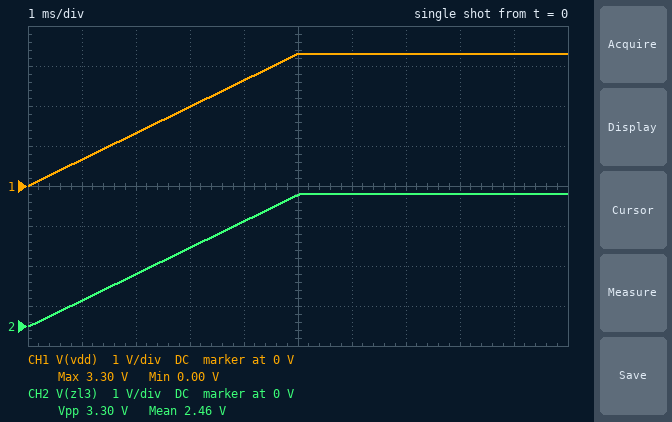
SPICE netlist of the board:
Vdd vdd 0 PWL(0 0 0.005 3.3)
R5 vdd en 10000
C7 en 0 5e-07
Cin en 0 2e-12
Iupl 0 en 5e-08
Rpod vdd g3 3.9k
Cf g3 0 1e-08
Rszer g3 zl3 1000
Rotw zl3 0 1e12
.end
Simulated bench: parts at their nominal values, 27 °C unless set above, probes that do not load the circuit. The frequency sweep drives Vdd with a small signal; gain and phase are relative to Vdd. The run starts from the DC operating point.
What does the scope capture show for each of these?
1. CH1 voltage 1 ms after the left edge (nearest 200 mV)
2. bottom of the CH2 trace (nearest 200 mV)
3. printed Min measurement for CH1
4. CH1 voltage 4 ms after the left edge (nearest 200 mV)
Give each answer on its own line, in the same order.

600 mV
0 V
0.00 V
2.6 V
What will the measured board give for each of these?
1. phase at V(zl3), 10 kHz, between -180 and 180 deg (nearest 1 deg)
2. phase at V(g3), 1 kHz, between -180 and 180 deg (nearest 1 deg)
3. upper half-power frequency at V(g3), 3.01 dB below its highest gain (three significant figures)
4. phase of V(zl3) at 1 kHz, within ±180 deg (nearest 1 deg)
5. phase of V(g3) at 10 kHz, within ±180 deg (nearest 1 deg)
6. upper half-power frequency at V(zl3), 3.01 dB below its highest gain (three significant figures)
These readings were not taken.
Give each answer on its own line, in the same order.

-68 deg
-14 deg
4.08 kHz
-14 deg
-68 deg
4.08 kHz
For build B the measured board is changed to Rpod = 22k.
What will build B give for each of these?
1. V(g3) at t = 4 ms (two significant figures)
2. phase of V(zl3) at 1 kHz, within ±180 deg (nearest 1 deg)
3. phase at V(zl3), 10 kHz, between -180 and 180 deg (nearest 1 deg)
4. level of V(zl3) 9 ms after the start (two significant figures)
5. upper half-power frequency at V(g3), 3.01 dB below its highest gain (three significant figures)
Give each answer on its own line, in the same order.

2.5 V
-54 deg
-86 deg
3.3 V
723 Hz
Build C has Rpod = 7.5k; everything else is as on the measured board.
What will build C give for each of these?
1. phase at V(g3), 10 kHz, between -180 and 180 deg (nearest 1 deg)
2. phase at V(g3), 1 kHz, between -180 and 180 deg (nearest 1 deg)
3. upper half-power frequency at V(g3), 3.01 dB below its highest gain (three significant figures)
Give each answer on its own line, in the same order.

-78 deg
-25 deg
2.12 kHz
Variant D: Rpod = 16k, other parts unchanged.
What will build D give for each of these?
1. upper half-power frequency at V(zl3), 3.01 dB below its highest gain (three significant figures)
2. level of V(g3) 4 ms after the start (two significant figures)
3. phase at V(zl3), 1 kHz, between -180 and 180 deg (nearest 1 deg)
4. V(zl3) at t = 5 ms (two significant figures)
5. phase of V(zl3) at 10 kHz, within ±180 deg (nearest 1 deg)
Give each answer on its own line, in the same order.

995 Hz
2.5 V
-45 deg
3.2 V
-84 deg
